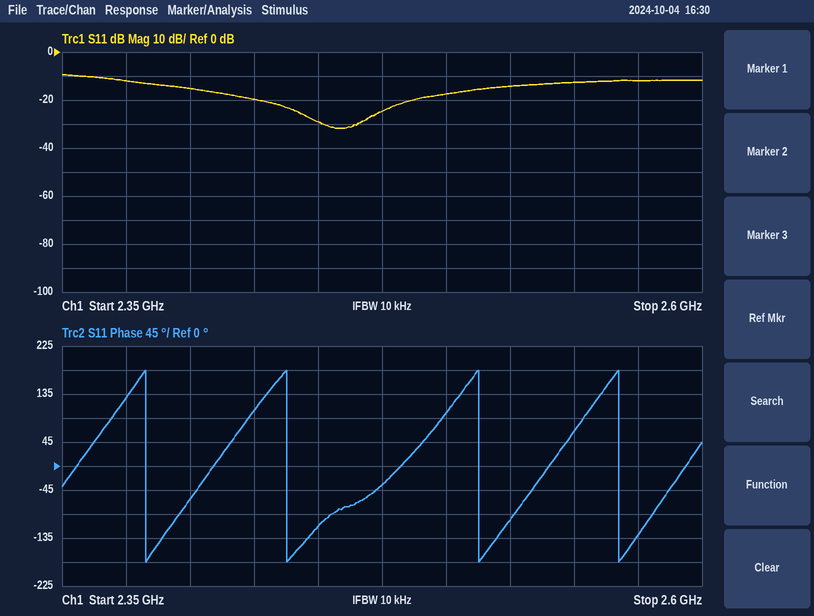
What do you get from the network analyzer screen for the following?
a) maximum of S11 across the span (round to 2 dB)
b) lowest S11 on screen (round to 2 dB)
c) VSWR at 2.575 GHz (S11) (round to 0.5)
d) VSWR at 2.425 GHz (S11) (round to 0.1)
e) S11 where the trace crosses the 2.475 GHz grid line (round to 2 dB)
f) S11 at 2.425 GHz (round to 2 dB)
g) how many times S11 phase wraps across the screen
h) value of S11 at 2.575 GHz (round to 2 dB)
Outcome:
-10 dB
-32 dB
1.5
1.2
-24 dB
-20 dB
4
-12 dB
